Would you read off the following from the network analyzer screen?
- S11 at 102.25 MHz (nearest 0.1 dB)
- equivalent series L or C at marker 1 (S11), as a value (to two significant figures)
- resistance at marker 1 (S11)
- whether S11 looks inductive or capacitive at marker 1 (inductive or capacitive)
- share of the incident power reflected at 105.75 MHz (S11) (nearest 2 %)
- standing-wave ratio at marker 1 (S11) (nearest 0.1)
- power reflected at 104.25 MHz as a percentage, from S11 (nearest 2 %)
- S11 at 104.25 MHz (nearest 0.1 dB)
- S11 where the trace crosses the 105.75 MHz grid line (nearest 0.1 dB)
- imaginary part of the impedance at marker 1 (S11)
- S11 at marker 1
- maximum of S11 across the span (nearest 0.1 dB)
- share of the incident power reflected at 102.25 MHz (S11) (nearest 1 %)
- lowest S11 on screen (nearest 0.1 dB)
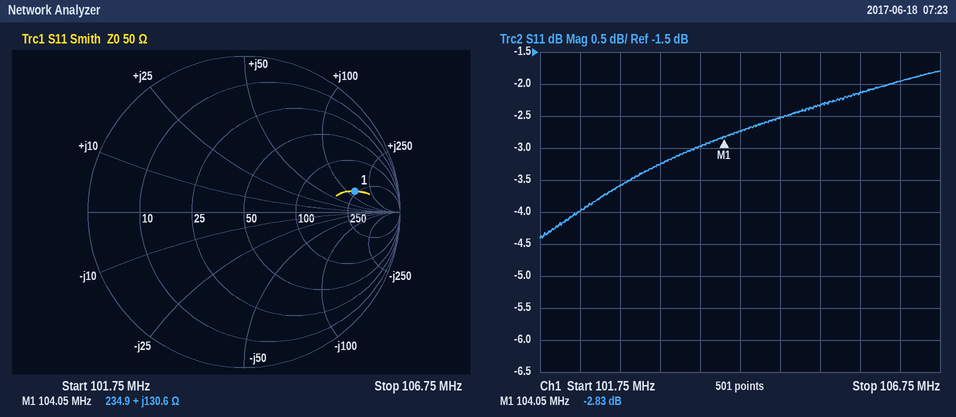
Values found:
-4.0 dB
200 nH
234.9 Ω
inductive
62 %
6.2
54 %
-2.7 dB
-2.1 dB
+130.6 Ω
-2.83 dB
-1.8 dB
40 %
-4.4 dB
